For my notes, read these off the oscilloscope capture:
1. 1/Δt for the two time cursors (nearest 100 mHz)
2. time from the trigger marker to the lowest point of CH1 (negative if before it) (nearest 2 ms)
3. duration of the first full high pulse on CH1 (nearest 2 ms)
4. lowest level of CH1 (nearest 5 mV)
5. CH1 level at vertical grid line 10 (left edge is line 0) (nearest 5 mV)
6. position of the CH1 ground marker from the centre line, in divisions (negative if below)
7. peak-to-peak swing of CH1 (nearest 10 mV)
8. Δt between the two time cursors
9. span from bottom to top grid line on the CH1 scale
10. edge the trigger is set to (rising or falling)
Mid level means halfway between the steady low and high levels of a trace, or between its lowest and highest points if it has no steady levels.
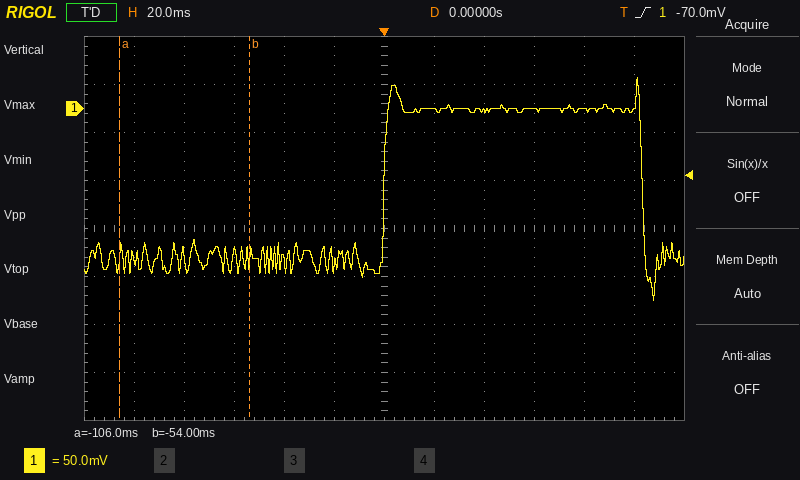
19.2 Hz
+108 ms
104 ms
-200 mV
0 mV
+2.5 div
230 mV
52 ms
400 mV
rising
